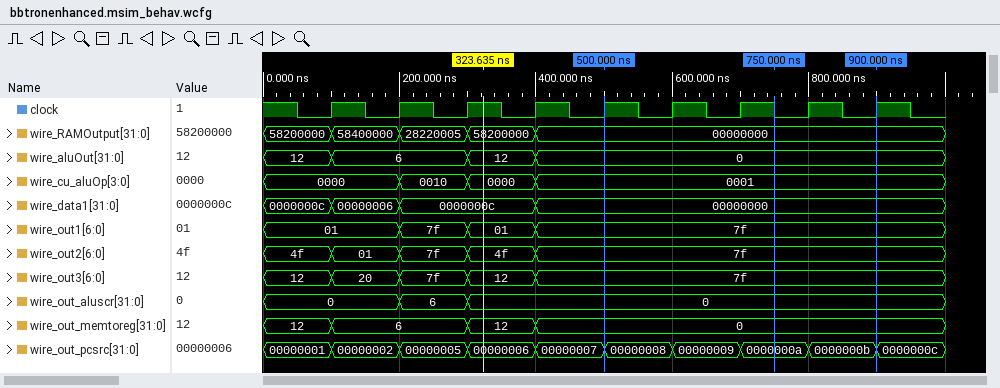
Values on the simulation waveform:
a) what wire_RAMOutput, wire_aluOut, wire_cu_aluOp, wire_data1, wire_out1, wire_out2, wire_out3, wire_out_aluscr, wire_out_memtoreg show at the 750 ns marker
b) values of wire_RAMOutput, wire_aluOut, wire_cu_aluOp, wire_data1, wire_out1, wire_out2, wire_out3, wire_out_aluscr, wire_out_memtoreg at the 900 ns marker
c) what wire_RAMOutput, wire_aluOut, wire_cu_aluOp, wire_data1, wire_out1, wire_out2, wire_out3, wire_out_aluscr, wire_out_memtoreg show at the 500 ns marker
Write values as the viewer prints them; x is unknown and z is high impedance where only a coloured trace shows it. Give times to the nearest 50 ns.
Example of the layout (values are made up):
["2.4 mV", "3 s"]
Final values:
["wire_RAMOutput=00000000, wire_aluOut=0, wire_cu_aluOp=0001, wire_data1=00000000, wire_out1=7f, wire_out2=7f, wire_out3=7f, wire_out_aluscr=0, wire_out_memtoreg=0", "wire_RAMOutput=00000000, wire_aluOut=0, wire_cu_aluOp=0001, wire_data1=00000000, wire_out1=7f, wire_out2=7f, wire_out3=7f, wire_out_aluscr=0, wire_out_memtoreg=0", "wire_RAMOutput=00000000, wire_aluOut=0, wire_cu_aluOp=0001, wire_data1=00000000, wire_out1=7f, wire_out2=7f, wire_out3=7f, wire_out_aluscr=0, wire_out_memtoreg=0"]
